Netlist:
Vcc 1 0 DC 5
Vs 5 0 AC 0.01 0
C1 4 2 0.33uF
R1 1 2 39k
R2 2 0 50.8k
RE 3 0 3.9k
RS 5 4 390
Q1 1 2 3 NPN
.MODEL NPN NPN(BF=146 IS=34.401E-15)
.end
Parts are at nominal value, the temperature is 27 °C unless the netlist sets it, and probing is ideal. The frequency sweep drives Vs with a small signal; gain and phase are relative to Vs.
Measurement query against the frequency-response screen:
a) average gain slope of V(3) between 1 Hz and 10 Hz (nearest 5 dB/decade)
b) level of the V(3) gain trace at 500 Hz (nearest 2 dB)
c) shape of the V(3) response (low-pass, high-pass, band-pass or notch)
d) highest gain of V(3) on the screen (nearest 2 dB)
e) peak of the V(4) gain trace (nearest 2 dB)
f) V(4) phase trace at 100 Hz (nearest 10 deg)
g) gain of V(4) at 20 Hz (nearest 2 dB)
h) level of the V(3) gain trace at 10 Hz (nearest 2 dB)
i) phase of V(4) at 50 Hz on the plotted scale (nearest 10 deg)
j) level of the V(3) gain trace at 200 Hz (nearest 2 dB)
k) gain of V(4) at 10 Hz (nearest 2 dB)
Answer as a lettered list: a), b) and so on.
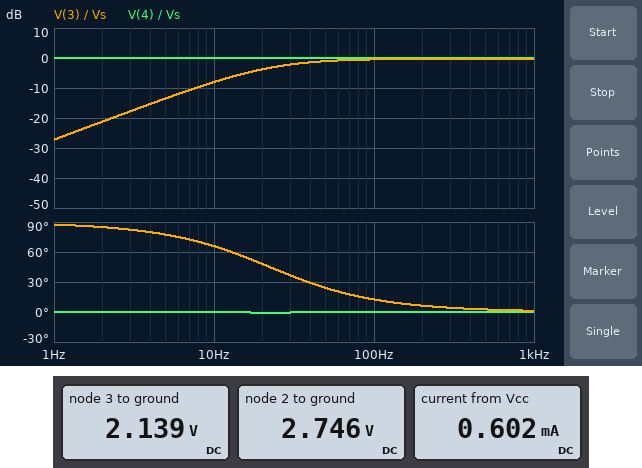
a) 20 dB/decade
b) 0 dB
c) high-pass
d) 0 dB
e) 0 dB
f) 0 deg
g) 0 dB
h) -8 dB
i) 0 deg
j) 0 dB
k) 0 dB
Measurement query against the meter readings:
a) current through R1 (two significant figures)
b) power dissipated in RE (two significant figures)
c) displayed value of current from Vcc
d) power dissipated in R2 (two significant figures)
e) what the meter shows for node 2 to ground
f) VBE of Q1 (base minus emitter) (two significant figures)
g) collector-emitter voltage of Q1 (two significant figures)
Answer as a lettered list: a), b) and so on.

a) 58 µA
b) 1.2 mW
c) 0.602 mA
d) 150 µW
e) 2.746 V
f) 610 mV
g) 2.9 V
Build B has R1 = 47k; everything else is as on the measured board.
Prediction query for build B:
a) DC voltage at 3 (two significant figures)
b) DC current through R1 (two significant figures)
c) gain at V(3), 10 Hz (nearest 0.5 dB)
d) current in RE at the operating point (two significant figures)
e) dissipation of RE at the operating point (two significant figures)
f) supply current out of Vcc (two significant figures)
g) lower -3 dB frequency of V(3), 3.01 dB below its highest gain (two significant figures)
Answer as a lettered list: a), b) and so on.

a) 1.9 V
b) 53 µA
c) -7.5 dB
d) 490 µA
e) 940 µW
f) 540 µA
g) 20 Hz
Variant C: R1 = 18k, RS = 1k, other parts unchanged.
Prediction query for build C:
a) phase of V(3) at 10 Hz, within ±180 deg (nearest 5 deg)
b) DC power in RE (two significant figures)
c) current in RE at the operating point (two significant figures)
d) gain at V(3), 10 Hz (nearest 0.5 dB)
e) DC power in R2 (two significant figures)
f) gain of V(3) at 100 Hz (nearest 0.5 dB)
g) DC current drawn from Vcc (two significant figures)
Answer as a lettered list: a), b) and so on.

a) 75 deg
b) 2.3 mW
c) 770 µA
d) -12.0 dB
e) 260 µW
f) -1.0 dB
g) 840 µA
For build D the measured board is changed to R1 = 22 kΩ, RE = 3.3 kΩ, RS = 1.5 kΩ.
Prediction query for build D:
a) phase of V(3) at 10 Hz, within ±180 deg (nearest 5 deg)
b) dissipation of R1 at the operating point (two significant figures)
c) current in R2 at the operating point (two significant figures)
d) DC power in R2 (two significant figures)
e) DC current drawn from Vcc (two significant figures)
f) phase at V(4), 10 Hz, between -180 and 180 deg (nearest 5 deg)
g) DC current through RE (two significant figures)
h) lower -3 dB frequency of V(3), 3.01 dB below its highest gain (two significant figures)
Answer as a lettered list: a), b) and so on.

a) 70 deg
b) 120 µW
c) 67 µA
d) 230 µW
e) 910 µA
f) 0 deg
g) 840 µA
h) 29 Hz
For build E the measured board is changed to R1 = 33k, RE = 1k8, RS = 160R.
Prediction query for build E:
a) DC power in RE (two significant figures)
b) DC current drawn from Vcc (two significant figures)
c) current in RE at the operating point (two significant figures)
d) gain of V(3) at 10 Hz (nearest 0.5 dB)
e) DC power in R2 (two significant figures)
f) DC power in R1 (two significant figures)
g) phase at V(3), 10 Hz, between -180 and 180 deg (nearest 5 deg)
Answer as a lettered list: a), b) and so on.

a) 2.8 mW
b) 1.3 mA
c) 1.2 mA
d) -9.0 dB
e) 160 µW
f) 140 µW
g) 70 deg
